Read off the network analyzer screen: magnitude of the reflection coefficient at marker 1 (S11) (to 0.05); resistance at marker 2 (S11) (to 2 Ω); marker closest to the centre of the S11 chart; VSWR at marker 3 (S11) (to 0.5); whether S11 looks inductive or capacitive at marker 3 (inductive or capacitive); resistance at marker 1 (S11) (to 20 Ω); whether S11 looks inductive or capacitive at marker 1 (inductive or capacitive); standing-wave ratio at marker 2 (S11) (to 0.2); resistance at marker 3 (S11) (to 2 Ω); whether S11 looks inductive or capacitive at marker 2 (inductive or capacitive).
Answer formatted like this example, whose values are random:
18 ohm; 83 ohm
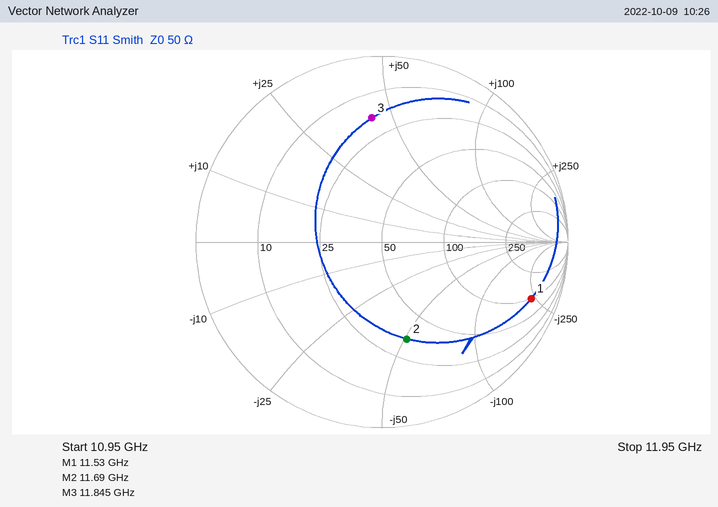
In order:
0.85; 34 Ω; marker 2; 5.0; inductive; 100 Ω; capacitive; 3.4; 18 Ω; capacitive
